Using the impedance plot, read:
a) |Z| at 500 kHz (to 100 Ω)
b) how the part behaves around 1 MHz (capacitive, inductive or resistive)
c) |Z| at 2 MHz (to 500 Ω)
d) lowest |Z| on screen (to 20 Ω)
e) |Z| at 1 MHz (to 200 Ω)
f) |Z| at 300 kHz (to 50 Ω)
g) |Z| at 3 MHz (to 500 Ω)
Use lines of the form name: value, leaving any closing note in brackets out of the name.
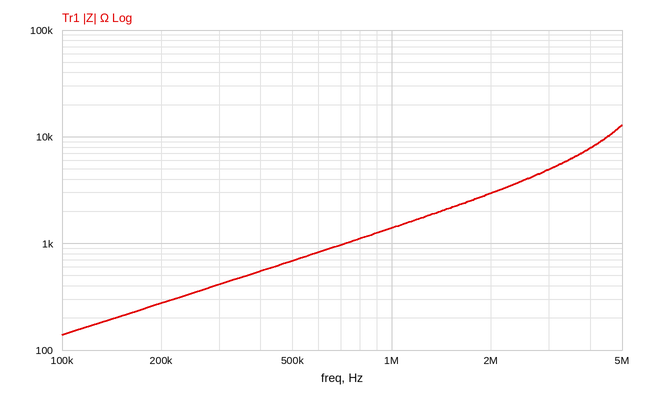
|Z| at 500 kHz: 700 Ω
how the part behaves around 1 MHz: inductive
|Z| at 2 MHz: 3.0 kΩ
lowest |Z| on screen: 140 Ω
|Z| at 1 MHz: 1.4 kΩ
|Z| at 300 kHz: 400 Ω
|Z| at 3 MHz: 5.0 kΩ
